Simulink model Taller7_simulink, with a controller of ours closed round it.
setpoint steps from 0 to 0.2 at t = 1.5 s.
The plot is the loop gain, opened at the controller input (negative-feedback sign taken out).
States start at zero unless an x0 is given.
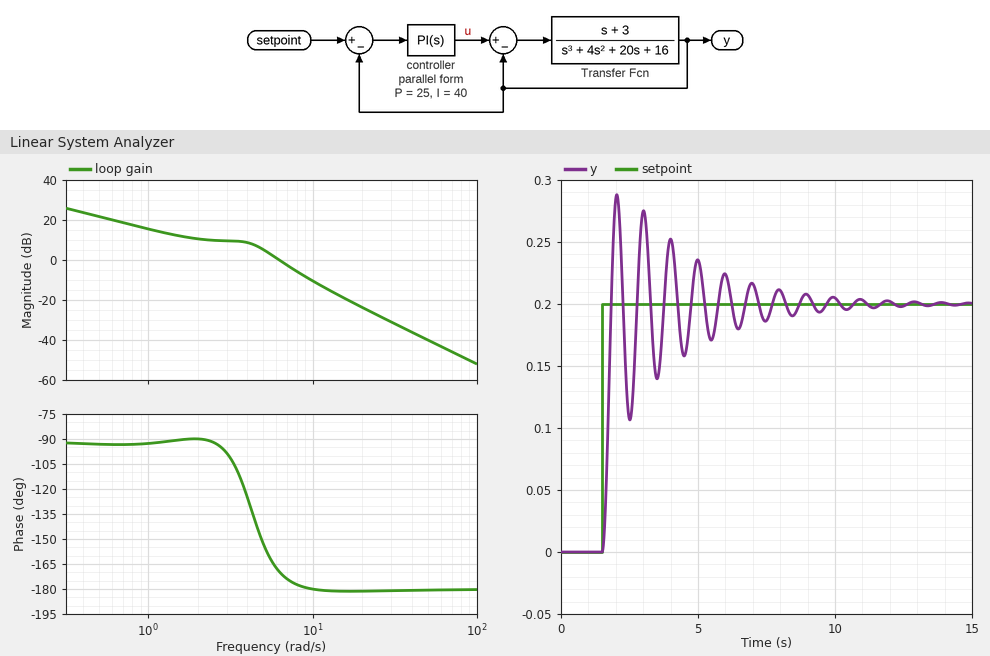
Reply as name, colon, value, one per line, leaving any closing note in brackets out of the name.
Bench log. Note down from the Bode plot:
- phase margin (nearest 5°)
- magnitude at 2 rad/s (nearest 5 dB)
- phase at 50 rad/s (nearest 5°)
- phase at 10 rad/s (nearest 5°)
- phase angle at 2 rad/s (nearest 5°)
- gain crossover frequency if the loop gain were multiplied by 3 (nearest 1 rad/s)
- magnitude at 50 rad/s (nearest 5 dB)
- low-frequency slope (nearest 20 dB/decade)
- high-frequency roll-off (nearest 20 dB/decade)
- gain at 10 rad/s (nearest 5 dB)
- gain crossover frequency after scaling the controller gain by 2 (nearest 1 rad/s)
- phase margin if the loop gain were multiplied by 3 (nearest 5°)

phase margin: 10°
magnitude at 2 rad/s: 10 dB
phase at 50 rad/s: -180°
phase at 10 rad/s: -180°
phase angle at 2 rad/s: -90°
gain crossover frequency if the loop gain were multiplied by 3: 10 rad/s
magnitude at 50 rad/s: -40 dB
low-frequency slope: -20 dB/decade
high-frequency roll-off: -40 dB/decade
gain at 10 rad/s: -10 dB
gain crossover frequency after scaling the controller gain by 2: 8 rad/s
phase margin if the loop gain were multiplied by 3: 0°
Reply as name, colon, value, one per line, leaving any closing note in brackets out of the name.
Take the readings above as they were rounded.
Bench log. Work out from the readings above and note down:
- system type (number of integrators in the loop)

system type: 1
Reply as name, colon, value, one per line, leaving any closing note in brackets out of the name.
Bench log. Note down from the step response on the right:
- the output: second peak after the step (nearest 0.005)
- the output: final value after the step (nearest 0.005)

the output: second peak after the step: 0.275
the output: final value after the step: 0.200
